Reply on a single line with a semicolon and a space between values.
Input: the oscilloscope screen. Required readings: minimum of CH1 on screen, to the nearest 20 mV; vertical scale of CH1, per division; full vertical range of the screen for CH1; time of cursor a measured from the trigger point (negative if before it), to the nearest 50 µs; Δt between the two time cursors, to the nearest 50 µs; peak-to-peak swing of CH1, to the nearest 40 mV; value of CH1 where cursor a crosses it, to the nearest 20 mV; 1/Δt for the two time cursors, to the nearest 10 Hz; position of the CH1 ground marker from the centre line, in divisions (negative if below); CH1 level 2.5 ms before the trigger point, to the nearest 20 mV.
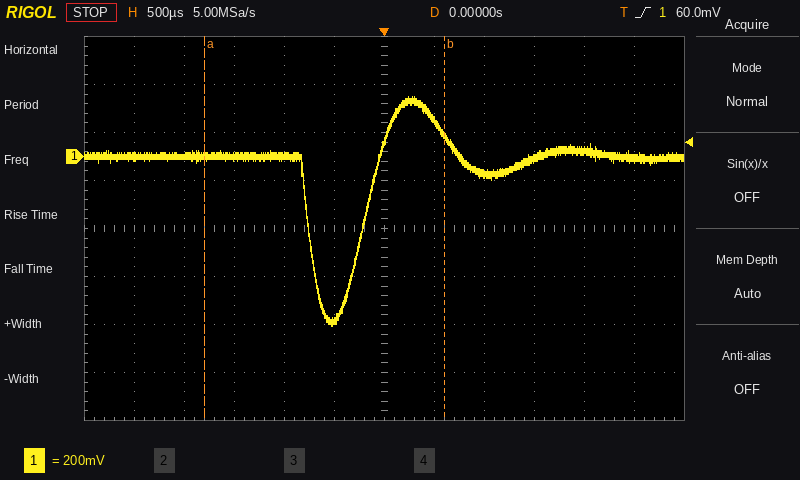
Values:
-700 mV; 200 mV; 1.6 V; -1.80 ms; 2.40 ms; 960 mV; 0 mV; 420 Hz; +1.5 div; 0 mV
